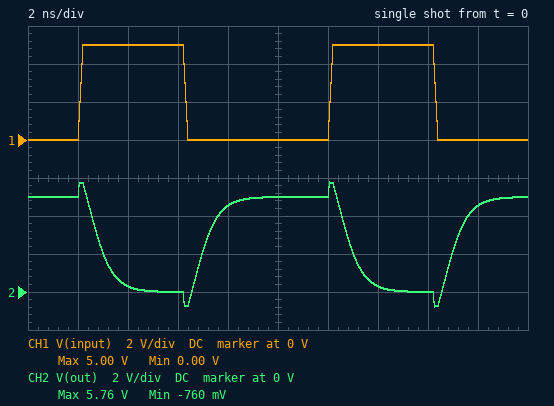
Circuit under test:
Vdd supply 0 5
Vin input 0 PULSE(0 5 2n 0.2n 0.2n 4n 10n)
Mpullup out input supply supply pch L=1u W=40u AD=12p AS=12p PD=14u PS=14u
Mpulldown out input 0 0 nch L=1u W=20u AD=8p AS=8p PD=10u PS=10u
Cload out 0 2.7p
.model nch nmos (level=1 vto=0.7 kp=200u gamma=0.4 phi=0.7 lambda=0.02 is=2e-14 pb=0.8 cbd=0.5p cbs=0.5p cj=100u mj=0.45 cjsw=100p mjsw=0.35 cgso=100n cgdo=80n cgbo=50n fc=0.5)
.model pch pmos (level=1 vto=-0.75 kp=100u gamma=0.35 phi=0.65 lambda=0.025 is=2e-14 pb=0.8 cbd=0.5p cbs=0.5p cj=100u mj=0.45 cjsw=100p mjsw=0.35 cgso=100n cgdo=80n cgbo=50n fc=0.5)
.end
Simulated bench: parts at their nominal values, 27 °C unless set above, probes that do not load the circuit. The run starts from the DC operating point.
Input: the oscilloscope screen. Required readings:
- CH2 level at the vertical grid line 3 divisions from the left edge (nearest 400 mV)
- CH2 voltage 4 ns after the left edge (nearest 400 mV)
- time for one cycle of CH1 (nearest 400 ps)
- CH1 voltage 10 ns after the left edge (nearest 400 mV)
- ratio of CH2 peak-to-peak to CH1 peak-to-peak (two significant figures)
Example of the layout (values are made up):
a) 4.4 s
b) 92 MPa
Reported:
a) 0 V
b) 400 mV
c) 10.0 ns
d) 0 V
e) 1.3
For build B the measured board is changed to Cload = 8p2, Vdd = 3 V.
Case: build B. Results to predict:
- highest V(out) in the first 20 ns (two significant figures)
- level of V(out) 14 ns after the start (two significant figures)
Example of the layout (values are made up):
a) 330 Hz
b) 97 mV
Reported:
a) 3.8 V
b) 590 mV
